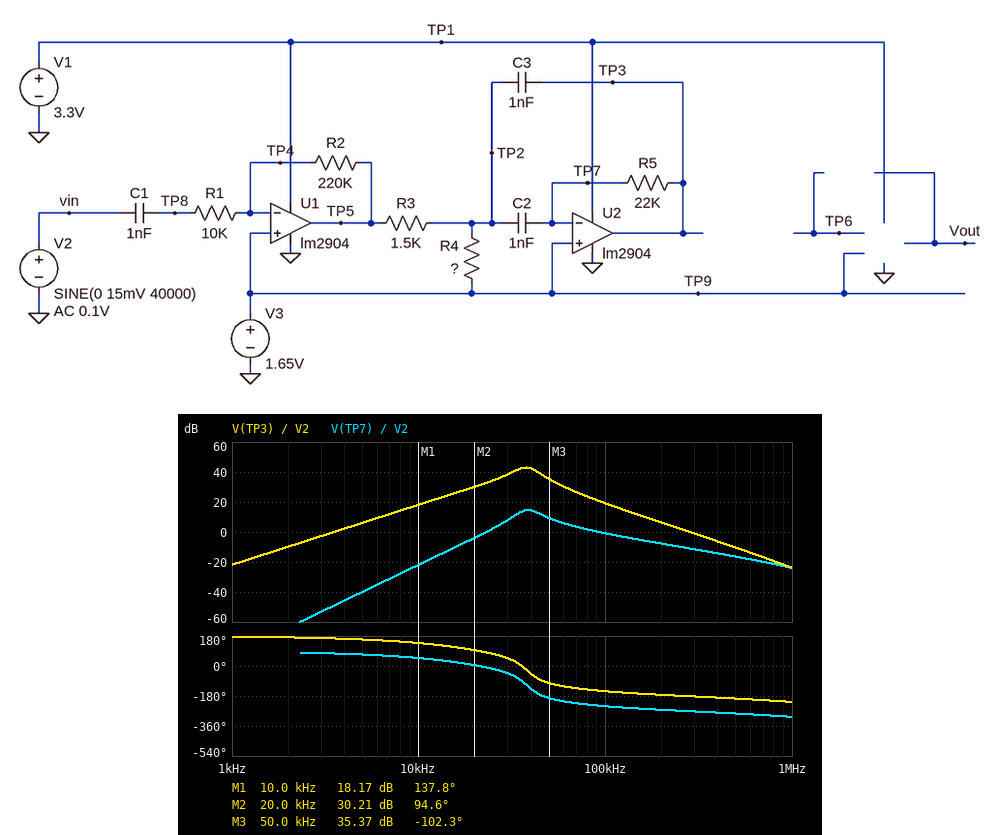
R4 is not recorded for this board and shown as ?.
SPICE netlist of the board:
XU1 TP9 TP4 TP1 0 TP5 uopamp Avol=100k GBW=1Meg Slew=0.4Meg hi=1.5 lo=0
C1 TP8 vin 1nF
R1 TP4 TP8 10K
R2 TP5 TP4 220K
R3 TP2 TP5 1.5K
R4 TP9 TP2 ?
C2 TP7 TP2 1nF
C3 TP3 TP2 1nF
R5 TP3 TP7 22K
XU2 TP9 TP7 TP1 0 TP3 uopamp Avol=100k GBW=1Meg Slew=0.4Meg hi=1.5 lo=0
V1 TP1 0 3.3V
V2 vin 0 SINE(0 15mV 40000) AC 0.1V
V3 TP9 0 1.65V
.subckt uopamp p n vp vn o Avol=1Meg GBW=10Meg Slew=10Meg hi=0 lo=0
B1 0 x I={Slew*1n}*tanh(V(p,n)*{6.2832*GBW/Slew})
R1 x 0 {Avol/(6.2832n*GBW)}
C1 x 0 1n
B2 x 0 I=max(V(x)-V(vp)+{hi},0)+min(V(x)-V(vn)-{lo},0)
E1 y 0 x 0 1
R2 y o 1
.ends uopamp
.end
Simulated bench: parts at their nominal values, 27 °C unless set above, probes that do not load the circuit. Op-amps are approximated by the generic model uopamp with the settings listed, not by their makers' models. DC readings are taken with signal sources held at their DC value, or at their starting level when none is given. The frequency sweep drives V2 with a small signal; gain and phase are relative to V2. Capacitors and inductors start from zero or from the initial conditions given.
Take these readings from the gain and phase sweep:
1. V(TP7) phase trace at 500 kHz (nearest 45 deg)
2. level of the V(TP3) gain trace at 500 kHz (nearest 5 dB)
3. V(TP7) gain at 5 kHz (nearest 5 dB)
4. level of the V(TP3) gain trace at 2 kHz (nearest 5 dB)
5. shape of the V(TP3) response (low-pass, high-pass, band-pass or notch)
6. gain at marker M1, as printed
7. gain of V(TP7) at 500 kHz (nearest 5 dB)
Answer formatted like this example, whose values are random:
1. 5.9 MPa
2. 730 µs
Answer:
1. -270 deg
2. -10 dB
3. -40 dB
4. -10 dB
5. band-pass
6. 18.17 dB
7. -15 dB
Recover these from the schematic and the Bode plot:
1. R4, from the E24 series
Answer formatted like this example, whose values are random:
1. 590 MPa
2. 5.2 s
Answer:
1. 1.1 kΩ
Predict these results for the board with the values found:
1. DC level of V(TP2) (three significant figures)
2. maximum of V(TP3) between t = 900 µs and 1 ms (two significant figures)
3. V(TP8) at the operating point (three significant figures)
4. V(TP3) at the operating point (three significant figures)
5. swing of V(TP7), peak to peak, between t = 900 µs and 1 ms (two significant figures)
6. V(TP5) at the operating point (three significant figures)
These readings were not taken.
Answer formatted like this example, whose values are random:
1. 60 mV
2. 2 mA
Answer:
1. 1.65 V
2. 1.8 V
3. 1.65 V
4. 1.65 V
5. 150 mV
6. 1.65 V
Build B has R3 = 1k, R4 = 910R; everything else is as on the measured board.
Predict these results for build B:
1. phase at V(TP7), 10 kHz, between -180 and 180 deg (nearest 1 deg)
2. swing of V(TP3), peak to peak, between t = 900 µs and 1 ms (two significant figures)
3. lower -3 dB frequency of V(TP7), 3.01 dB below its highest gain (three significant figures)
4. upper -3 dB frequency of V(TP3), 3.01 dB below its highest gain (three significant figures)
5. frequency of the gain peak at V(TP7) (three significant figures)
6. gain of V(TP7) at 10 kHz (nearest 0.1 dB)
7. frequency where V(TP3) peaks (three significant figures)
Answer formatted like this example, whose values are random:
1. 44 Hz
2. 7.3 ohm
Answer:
1. 49 deg
2. 590 mV
3. 37.8 kHz
4. 47.6 kHz
5. 42.8 kHz
6. -20.9 dB
7. 42.1 kHz
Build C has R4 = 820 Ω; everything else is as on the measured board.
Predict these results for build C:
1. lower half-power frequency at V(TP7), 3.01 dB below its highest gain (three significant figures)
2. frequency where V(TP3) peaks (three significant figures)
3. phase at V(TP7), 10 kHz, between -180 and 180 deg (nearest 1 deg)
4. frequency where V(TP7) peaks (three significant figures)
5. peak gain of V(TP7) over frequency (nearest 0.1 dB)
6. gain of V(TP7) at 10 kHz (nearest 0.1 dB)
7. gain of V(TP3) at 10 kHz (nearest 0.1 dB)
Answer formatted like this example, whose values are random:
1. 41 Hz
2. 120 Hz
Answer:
1. 36.1 kHz
2. 40.4 kHz
3. 49 deg
4. 41.2 kHz
5. 14.8 dB
6. -23.5 dB
7. 16.5 dB
